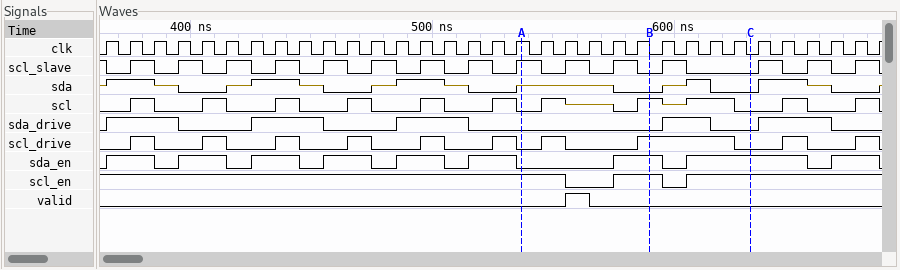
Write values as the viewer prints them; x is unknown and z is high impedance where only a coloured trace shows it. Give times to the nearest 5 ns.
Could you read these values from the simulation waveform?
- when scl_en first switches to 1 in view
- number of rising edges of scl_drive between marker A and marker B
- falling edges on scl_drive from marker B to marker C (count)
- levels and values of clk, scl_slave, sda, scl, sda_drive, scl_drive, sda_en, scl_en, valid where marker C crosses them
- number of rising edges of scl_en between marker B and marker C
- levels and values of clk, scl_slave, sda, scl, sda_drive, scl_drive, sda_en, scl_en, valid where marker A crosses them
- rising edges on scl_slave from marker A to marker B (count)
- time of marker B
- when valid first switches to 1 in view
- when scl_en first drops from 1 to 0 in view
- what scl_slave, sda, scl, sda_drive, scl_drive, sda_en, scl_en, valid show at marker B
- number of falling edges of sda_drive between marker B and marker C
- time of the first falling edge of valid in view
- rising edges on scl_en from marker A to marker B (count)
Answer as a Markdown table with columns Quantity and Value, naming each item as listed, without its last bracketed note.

| Quantity | Value |
|---|---|
| when scl_en first switches to 1 in view | 575 ns |
| number of rising edges of scl_drive between marker A and marker B | 2 |
| falling edges on scl_drive from marker B to marker C | 1 |
| levels and values of clk, scl_slave, sda, scl, sda_drive, scl_drive, sda_en, scl_en, valid where marker C crosses them | clk=0, scl_slave=0, sda=0, scl=0, sda_drive=0, scl_drive=0, sda_en=1, scl_en=1, valid=0 |
| number of rising edges of scl_en between marker B and marker C | 1 |
| levels and values of clk, scl_slave, sda, scl, sda_drive, scl_drive, sda_en, scl_en, valid where marker A crosses them | clk=1, scl_slave=1, sda=z, scl=0, sda_drive=0, scl_drive=0, sda_en=0, scl_en=1, valid=0 |
| rising edges on scl_slave from marker A to marker B | 2 |
| time of marker B | 590 ns |
| when valid first switches to 1 in view | 555 ns |
| when scl_en first drops from 1 to 0 in view | 555 ns |
| what scl_slave, sda, scl, sda_drive, scl_drive, sda_en, scl_en, valid show at marker B | scl_slave=0, sda=0, scl=1, sda_drive=0, scl_drive=1, sda_en=1, scl_en=1, valid=0 |
| number of falling edges of sda_drive between marker B and marker C | 1 |
| time of the first falling edge of valid in view | 565 ns |
| rising edges on scl_en from marker A to marker B | 1 |
